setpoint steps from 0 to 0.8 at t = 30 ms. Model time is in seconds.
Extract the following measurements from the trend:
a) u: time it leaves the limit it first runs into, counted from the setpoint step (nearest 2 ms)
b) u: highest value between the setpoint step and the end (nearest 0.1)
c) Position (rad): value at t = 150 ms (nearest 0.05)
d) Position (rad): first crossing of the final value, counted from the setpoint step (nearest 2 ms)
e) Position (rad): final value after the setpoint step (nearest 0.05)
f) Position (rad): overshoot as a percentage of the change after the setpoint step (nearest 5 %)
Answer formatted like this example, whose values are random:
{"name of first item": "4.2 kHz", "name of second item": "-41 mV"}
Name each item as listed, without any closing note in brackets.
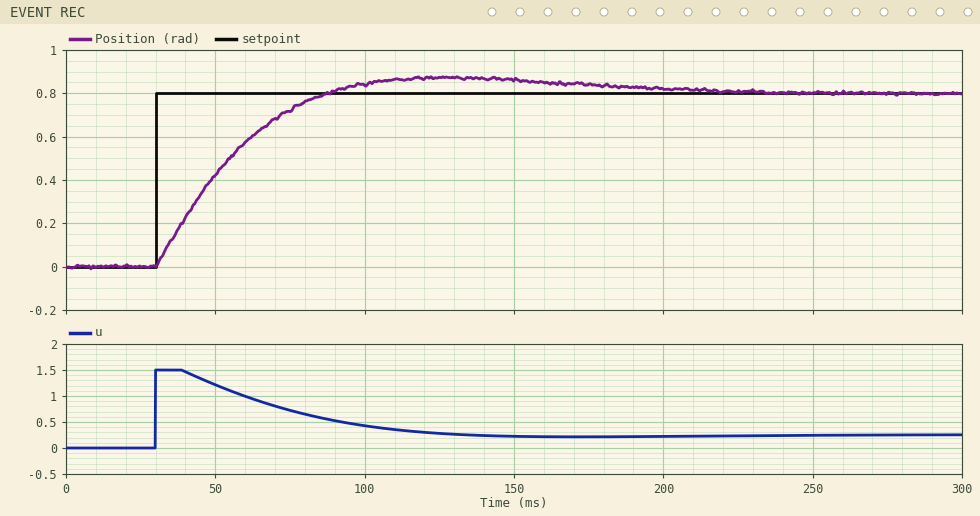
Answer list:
{"u: time it leaves the limit it first runs into, counted from the setpoint step": "10 ms", "u: highest value between the setpoint step and the end": "1.5", "Position (rad): value at t = 150 ms": "0.85", "Position (rad): first crossing of the final value, counted from the setpoint step": "58 ms", "Position (rad): final value after the setpoint step": "0.80", "Position (rad): overshoot as a percentage of the change after the setpoint step": "10 %"}
